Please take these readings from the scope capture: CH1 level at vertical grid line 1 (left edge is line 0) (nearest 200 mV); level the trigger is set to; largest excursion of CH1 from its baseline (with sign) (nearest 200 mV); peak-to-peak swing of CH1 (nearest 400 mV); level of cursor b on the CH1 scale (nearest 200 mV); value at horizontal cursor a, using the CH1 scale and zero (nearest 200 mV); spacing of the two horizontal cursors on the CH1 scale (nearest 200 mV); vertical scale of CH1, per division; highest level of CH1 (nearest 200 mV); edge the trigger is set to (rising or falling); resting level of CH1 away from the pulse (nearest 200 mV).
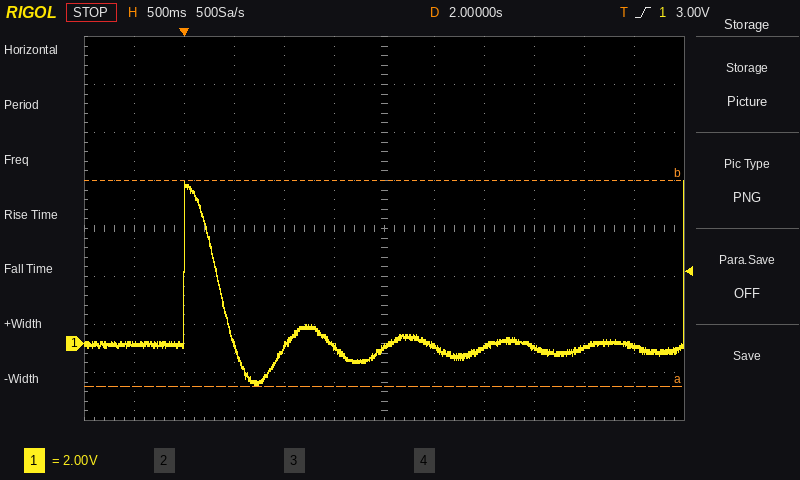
0.0 V
3.00 V
+6.8 V
8.4 V
6.8 V
-1.8 V
8.6 V
2 V
6.8 V
rising
0.0 V
